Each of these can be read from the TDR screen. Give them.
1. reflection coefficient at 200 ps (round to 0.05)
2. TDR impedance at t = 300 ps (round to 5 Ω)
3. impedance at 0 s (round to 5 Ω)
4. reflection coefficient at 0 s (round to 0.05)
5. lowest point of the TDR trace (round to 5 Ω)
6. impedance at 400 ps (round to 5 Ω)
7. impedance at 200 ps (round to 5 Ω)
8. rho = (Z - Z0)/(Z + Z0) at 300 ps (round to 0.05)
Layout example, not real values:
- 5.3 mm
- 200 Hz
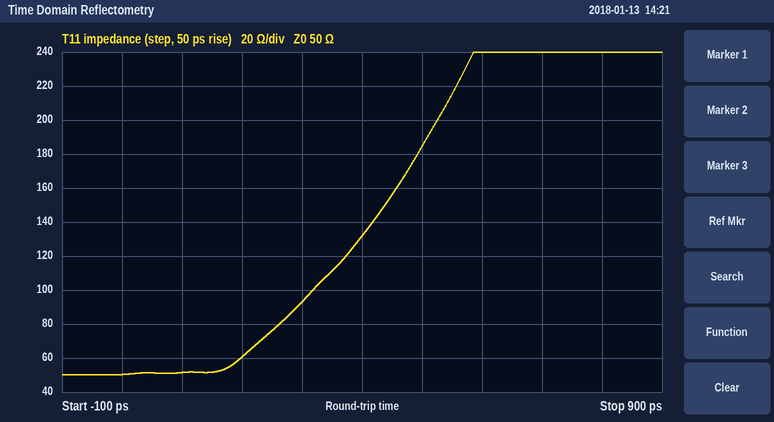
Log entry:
- +0.10
- 95 Ω
- 50 Ω
- 0.00
- 50 Ω
- 130 Ω
- 60 Ω
- +0.30
